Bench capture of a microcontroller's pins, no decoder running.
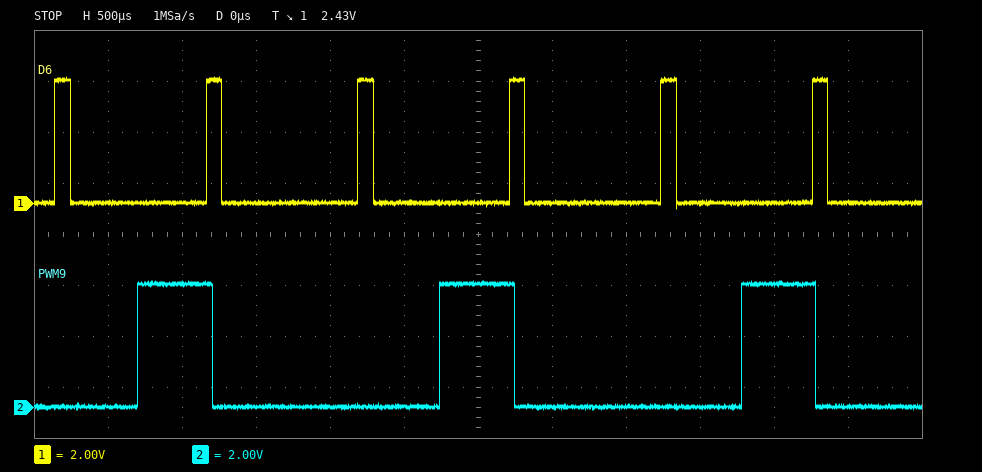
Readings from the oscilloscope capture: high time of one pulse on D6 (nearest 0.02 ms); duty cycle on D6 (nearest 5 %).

0.10 ms
10 %
